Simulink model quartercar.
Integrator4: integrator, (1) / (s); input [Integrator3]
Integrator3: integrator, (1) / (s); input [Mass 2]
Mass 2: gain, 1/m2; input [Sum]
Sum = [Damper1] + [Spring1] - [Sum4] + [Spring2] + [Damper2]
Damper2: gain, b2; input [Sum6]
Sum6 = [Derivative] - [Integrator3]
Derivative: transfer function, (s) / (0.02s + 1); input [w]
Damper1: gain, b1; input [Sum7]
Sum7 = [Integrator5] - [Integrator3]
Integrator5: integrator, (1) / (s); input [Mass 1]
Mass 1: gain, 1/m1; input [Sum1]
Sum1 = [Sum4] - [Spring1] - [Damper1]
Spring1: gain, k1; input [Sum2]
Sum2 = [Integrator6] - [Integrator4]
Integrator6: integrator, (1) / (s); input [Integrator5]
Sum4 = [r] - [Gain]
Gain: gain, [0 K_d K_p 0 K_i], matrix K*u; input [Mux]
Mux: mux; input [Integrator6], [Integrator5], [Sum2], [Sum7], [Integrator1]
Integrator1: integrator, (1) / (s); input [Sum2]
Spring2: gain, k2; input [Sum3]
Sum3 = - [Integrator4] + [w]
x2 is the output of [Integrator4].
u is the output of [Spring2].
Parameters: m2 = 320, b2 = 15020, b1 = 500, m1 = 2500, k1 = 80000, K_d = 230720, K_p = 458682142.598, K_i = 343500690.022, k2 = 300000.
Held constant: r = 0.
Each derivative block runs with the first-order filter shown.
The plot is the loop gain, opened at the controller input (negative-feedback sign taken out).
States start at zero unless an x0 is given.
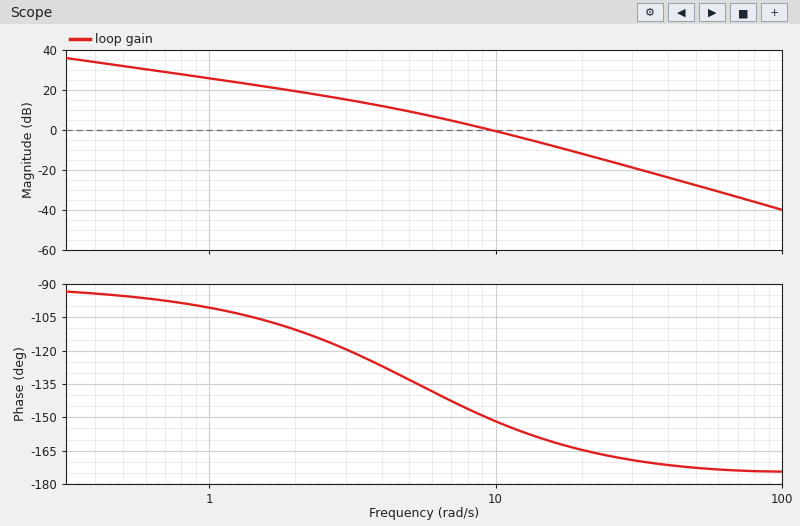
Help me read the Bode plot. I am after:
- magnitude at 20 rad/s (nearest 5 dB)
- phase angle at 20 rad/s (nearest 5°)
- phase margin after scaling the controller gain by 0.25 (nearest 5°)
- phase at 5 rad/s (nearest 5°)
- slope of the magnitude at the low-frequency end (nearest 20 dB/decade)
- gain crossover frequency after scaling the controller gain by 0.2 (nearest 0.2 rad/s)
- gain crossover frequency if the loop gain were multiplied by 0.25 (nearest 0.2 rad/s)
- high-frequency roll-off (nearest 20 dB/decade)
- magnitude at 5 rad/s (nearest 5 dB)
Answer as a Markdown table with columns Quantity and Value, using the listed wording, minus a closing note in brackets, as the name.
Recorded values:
| Quantity | Value |
|---|---|
| magnitude at 20 rad/s | -10 dB |
| phase angle at 20 rad/s | -165° |
| phase margin after scaling the controller gain by 0.25 | 55° |
| phase at 5 rad/s | -135° |
| slope of the magnitude at the low-frequency end | -20 dB/decade |
| gain crossover frequency after scaling the controller gain by 0.2 | 3.4 rad/s |
| gain crossover frequency if the loop gain were multiplied by 0.25 | 4.0 rad/s |
| high-frequency roll-off | -40 dB/decade |
| magnitude at 5 rad/s | 10 dB |
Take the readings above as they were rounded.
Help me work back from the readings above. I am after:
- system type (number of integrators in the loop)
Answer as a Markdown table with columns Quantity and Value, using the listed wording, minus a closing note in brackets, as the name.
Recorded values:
| Quantity | Value |
|---|---|
| system type | 1 |
